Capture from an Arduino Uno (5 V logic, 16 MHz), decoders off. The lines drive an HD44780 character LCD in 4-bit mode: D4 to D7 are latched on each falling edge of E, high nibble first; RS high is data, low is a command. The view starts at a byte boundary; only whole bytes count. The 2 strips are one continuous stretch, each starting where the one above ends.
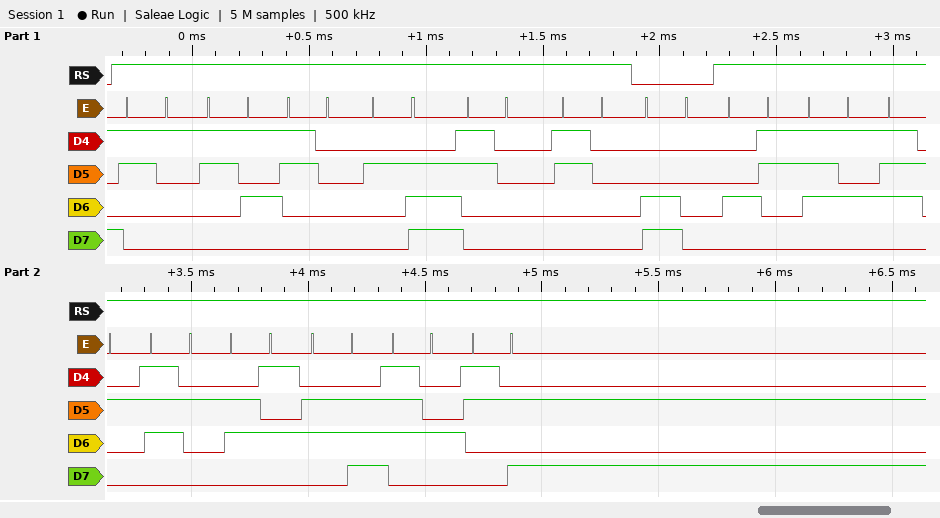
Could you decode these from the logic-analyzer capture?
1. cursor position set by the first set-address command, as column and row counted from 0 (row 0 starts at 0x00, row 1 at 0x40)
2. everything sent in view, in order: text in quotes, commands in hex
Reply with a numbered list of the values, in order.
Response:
1. column 0, row 1
2. "150.00" 0xC0 "Current:"
